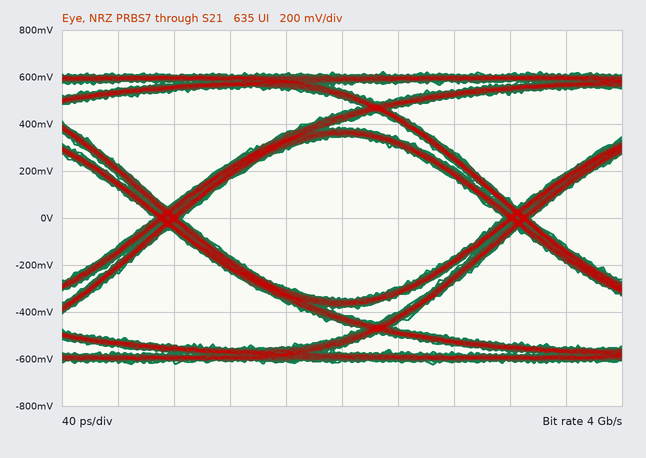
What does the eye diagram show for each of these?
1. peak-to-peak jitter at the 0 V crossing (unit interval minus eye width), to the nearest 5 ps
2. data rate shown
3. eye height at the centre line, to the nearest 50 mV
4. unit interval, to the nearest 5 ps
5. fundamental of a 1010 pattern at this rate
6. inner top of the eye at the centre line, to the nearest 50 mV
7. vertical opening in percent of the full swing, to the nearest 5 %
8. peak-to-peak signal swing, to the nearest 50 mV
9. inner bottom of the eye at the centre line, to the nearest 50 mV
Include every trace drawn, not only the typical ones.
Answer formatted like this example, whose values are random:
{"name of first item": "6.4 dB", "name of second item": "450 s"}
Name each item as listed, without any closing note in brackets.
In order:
{"peak-to-peak jitter at the 0 V crossing (unit interval minus eye width), to the nearest 5 ps": "20 ps", "data rate shown": "4 Gb/s", "eye height at the centre line, to the nearest 50 mV": "700 mV", "unit interval, to the nearest 5 ps": "250 ps", "fundamental of a 1010 pattern at this rate": "2 GHz", "inner top of the eye at the centre line, to the nearest 50 mV": "350 mV", "vertical opening in percent of the full swing, to the nearest 5 %": "55 %", "peak-to-peak signal swing, to the nearest 50 mV": "1.25 V", "inner bottom of the eye at the centre line, to the nearest 50 mV": "-350 mV"}
